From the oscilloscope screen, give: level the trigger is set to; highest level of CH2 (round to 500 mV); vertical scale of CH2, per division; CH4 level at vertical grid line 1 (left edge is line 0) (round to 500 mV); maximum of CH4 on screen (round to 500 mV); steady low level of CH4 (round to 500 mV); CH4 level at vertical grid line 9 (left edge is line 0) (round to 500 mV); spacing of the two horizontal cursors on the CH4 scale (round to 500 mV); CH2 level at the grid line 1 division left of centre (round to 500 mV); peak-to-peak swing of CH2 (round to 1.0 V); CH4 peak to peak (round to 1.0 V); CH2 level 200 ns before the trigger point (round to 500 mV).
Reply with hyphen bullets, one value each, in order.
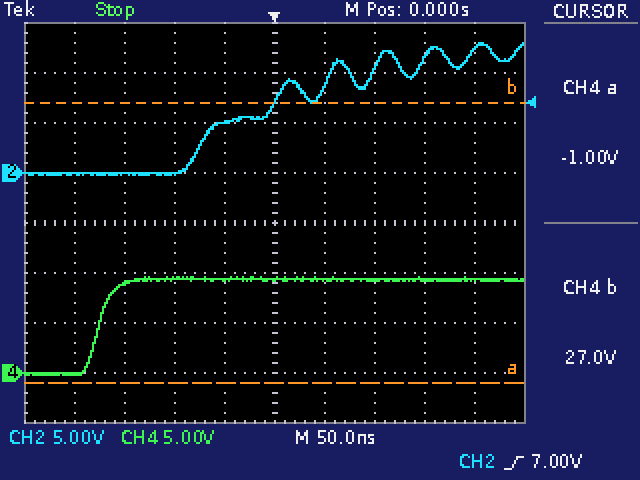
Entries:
- 7.00 V
- 13.0 V
- 5 V
- 0.0 V
- 9.5 V
- 0.0 V
- 9.5 V
- 28.0 V
- 5.0 V
- 13.0 V
- 10.0 V
- 0.0 V
